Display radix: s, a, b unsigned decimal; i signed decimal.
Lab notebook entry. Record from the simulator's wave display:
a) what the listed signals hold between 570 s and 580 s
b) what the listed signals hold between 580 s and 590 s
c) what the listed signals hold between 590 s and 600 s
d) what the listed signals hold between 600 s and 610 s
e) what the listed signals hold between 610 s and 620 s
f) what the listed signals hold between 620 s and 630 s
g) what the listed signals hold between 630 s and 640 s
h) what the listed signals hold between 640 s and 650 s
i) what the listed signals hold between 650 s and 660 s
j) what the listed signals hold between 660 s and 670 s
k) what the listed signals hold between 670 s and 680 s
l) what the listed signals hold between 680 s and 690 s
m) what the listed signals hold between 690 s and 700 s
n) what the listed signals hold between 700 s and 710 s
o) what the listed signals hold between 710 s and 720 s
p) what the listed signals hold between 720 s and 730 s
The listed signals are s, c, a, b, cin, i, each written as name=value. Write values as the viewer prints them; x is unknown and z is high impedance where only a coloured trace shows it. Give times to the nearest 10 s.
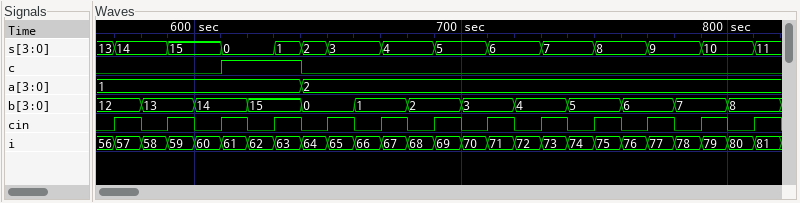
s=14, c=0, a=1, b=12, cin=1, i=57
s=14, c=0, a=1, b=13, cin=0, i=58
s=15, c=0, a=1, b=13, cin=1, i=59
s=15, c=0, a=1, b=14, cin=0, i=60
s=0, c=1, a=1, b=14, cin=1, i=61
s=0, c=1, a=1, b=15, cin=0, i=62
s=1, c=1, a=1, b=15, cin=1, i=63
s=2, c=0, a=2, b=0, cin=0, i=64
s=3, c=0, a=2, b=0, cin=1, i=65
s=3, c=0, a=2, b=1, cin=0, i=66
s=4, c=0, a=2, b=1, cin=1, i=67
s=4, c=0, a=2, b=2, cin=0, i=68
s=5, c=0, a=2, b=2, cin=1, i=69
s=5, c=0, a=2, b=3, cin=0, i=70
s=6, c=0, a=2, b=3, cin=1, i=71
s=6, c=0, a=2, b=4, cin=0, i=72
